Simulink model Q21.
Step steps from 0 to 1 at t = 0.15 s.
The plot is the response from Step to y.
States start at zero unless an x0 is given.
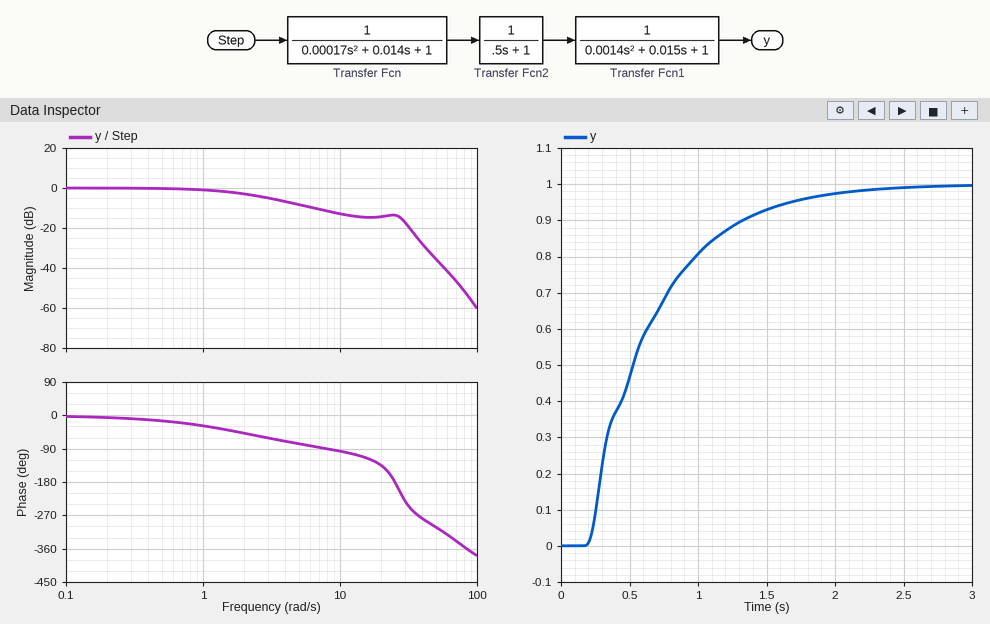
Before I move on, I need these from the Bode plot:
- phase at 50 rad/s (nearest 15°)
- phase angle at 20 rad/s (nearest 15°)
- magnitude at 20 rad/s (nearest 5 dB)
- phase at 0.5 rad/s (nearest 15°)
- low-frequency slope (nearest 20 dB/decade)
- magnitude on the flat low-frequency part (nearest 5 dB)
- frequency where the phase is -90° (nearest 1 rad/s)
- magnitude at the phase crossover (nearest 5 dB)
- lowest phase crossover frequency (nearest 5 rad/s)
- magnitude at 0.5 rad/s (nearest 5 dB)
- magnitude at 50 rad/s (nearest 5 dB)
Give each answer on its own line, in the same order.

-300°
-135°
-15 dB
-15°
0 dB/decade
0 dB
8 rad/s
-15 dB
25 rad/s
0 dB
-35 dB
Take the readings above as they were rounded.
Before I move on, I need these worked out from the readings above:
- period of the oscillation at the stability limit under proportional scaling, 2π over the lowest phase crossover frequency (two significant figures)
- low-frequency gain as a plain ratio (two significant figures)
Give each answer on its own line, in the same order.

0.25 s
1.0
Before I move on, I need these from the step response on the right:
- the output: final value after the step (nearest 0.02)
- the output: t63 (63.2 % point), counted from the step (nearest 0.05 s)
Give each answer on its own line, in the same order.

1.00
0.55 s
